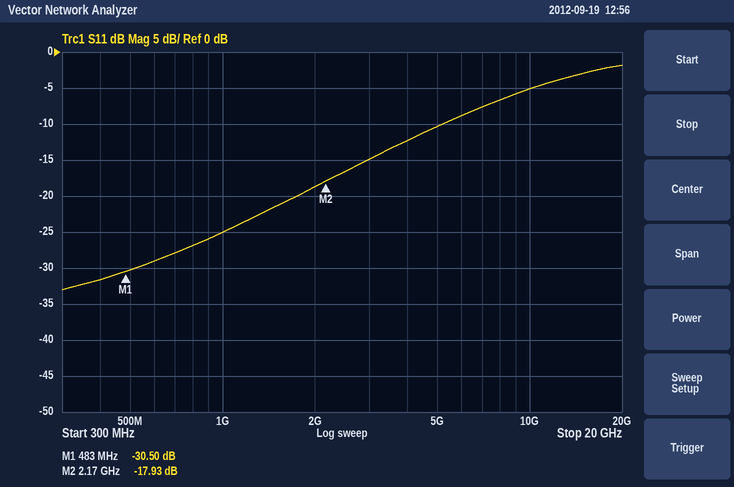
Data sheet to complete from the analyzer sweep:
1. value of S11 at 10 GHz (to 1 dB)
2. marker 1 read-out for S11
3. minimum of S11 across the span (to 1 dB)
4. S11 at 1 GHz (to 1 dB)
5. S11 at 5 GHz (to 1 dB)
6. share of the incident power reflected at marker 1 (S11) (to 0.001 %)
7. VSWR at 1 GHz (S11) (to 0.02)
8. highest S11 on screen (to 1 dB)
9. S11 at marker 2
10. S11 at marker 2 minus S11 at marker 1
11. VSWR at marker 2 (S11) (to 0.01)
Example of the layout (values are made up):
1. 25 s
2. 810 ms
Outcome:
1. -5 dB
2. -30.50 dB
3. -33 dB
4. -25 dB
5. -10 dB
6. 0.089 %
7. 1.12
8. -2 dB
9. -17.93 dB
10. 12.57 dB
11. 1.29
